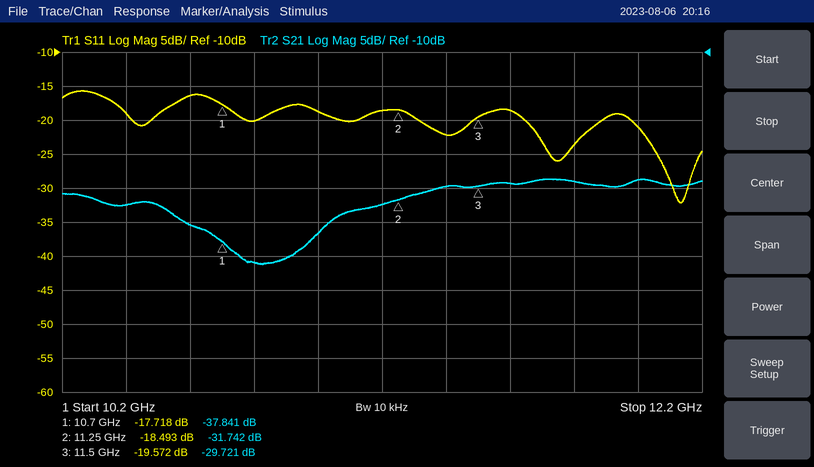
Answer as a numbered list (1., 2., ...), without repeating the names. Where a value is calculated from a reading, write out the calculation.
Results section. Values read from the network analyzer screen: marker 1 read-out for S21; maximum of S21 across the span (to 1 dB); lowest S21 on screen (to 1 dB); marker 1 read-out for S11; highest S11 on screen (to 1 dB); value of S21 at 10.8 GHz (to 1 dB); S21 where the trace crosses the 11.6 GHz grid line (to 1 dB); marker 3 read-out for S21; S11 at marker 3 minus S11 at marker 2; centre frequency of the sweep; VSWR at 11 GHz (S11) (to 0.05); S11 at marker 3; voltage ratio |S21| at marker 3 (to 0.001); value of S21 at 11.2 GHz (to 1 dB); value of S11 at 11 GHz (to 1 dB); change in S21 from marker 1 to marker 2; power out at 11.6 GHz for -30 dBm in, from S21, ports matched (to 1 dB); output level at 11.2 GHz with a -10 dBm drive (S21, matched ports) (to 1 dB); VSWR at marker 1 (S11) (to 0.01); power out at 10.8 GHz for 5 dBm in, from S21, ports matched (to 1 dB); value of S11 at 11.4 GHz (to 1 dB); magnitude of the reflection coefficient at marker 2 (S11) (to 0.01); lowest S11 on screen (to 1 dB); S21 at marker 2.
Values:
1. -37.841 dB
2. -29 dB
3. -41 dB
4. -17.718 dB
5. -16 dB
6. -41 dB
7. -29 dB
8. -29.721 dB
9. -19.572 − (-18.493) = -1.079 dB
10. 11.2 GHz
11. |Γ| = 10^(-19/20) = 0.1122; VSWR = (1 + 0.1122)/(1 − 0.1122) ≈ 1.25
12. -19.572 dB
13. 10^(-29.721/20) ≈ 0.033
14. -32 dB
15. -19 dB
16. -31.742 − (-37.841) = 6.099 dB
17. -30 dBm + (-29 dB) = -59 dBm
18. -10 dBm + (-32 dB) = -42 dBm
19. (1 + 0.1300)/(1 − 0.1300) ≈ 1.30
20. 5 dBm + (-41 dB) = -36 dBm
21. -22 dB
22. 10^(-18.493/20) ≈ 0.12
23. -32 dB
24. -31.742 dB
